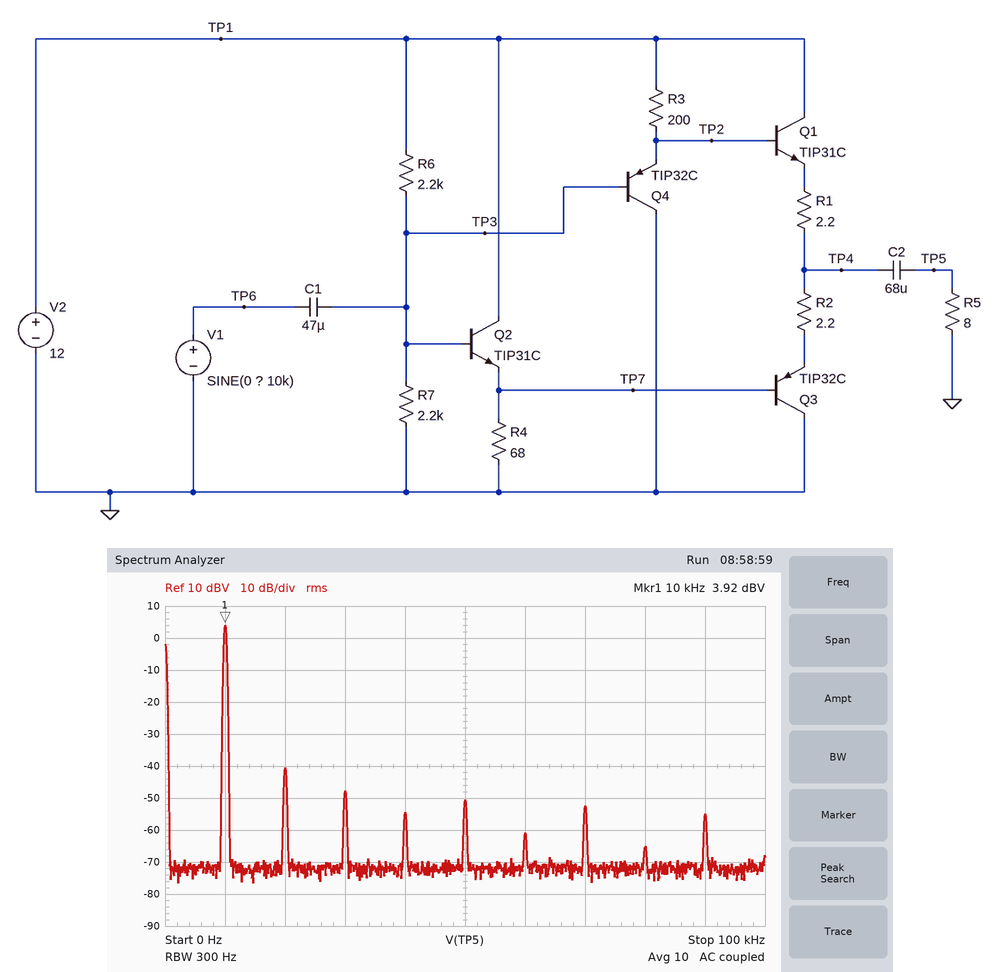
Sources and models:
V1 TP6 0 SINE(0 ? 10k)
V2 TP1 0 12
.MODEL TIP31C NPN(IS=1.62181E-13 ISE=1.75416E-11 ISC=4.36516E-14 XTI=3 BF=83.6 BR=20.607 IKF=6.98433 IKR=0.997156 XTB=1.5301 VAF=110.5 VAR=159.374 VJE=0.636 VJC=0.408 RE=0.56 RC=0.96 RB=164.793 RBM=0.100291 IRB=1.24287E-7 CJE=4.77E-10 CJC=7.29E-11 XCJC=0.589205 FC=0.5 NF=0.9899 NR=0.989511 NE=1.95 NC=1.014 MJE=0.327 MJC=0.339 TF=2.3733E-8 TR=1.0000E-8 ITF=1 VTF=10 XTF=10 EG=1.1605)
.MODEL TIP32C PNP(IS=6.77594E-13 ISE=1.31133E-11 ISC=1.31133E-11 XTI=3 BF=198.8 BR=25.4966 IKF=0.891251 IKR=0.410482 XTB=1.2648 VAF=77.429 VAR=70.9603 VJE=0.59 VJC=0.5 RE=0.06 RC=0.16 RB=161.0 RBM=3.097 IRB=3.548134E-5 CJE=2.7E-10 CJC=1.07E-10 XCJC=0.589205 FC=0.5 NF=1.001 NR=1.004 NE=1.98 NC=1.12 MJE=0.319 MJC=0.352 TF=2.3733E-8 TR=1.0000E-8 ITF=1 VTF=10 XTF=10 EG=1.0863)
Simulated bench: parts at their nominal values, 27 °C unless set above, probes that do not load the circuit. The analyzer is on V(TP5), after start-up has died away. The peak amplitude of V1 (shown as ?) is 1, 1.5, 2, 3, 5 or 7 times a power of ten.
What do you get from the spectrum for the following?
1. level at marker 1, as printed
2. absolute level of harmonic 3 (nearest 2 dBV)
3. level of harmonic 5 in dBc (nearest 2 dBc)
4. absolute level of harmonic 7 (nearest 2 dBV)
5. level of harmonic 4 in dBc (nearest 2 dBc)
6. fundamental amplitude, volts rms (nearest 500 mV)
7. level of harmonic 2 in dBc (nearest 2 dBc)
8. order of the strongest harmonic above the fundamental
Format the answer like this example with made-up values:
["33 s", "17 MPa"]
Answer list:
["3.92 dBV", "-48 dBV", "-54 dBc", "-52 dBV", "-58 dBc", "1.5 V", "-44 dBc", "2"]
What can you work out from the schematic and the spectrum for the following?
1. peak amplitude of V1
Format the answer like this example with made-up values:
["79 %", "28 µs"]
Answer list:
["3 V"]
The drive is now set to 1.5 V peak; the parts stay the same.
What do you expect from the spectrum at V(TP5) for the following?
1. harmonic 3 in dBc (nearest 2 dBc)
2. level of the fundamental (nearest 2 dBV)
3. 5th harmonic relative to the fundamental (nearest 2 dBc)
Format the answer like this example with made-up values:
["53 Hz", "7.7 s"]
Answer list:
["-44 dBc", "-2 dBV", "-48 dBc"]
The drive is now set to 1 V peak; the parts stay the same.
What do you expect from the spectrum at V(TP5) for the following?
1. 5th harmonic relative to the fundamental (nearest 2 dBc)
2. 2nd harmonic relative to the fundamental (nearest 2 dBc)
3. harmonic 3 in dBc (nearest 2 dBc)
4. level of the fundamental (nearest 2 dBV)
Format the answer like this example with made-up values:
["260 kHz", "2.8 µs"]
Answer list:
["-50 dBc", "-46 dBc", "-40 dBc", "-6 dBV"]
